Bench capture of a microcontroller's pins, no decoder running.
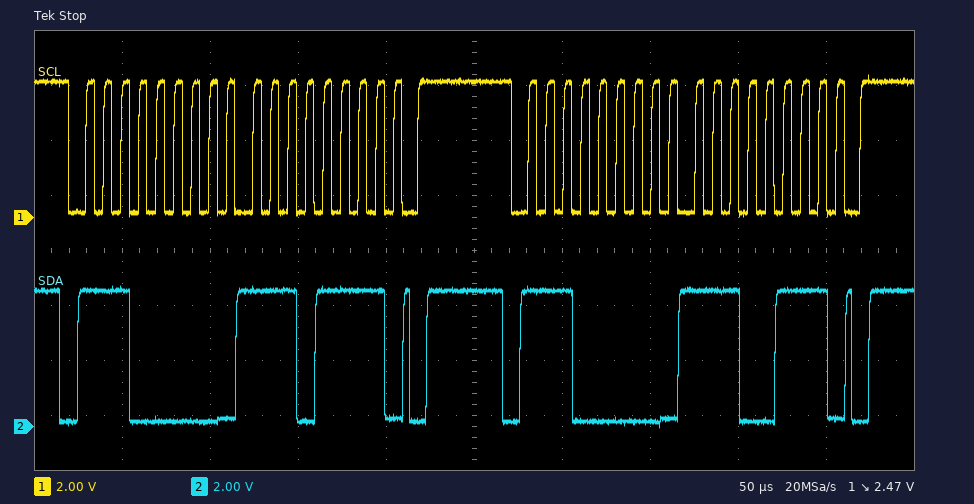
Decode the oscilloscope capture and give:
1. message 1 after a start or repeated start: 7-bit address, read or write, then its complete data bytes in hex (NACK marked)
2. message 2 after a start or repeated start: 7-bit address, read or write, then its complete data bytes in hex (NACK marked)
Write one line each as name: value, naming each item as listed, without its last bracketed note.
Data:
message 1 after a start or repeated start: 7-bit address, read or write, then its complete data bytes in hex: 0x70 write: EF
message 2 after a start or repeated start: 7-bit address, read or write, then its complete data bytes in hex: 0x70 write: E7
